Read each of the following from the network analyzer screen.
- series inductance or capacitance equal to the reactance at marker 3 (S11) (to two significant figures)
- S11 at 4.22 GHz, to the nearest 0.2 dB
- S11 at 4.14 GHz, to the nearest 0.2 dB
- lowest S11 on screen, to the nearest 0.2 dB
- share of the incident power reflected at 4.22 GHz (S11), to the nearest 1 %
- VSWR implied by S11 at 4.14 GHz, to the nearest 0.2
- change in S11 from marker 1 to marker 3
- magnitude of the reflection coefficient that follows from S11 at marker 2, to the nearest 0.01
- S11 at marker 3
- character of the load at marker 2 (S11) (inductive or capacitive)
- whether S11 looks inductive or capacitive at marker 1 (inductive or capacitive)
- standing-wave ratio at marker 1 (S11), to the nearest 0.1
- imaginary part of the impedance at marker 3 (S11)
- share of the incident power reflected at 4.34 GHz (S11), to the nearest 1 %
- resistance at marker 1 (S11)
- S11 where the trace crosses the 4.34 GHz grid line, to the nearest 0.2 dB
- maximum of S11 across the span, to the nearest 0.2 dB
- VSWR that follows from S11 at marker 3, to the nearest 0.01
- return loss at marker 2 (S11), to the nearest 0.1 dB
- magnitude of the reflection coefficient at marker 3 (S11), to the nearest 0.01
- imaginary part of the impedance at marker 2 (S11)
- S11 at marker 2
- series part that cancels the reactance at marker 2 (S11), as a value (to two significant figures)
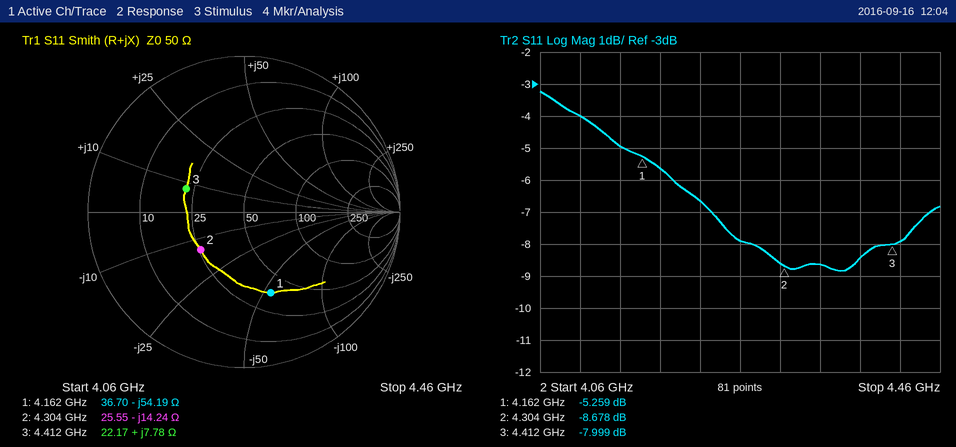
280 pH
-6.6 dB
-5.0 dB
-8.8 dB
22 %
3.6
-2.740 dB
0.37
-7.999 dB
capacitive
capacitive
3.4
+7.78 Ω
14 %
36.70 Ω
-8.6 dB
-3.2 dB
2.32
8.7 dB
0.40
-14.24 Ω
-8.678 dB
530 pH
